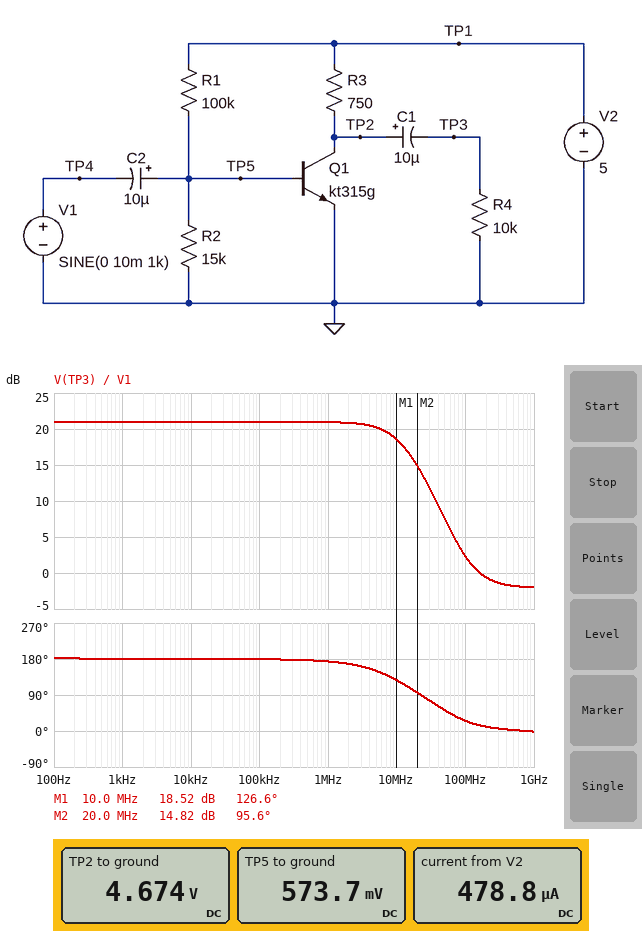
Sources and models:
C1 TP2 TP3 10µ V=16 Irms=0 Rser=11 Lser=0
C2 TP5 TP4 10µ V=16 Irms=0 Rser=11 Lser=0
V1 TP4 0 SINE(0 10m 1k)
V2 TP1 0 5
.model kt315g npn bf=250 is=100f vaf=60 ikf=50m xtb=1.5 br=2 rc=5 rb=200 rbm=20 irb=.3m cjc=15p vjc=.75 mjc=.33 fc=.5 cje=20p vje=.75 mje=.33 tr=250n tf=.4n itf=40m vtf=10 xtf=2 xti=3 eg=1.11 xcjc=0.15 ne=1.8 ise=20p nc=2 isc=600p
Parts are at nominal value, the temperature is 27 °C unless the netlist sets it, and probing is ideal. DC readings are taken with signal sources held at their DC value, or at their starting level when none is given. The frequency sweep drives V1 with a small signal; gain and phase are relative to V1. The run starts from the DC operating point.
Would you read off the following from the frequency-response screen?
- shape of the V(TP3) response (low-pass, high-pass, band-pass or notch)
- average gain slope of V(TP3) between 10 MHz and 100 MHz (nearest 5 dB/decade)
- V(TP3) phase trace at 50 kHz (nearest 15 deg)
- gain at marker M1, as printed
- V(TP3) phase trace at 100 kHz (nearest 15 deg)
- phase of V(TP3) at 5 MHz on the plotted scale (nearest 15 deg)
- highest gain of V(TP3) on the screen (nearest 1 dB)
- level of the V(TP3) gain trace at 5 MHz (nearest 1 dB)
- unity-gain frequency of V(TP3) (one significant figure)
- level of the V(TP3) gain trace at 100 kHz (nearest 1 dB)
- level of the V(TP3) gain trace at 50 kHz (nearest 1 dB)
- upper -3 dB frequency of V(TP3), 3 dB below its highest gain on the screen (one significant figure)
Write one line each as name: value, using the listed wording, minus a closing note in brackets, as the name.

shape of the V(TP3) response: low-pass
average gain slope of V(TP3) between 10 MHz and 100 MHz: -15 dB/decade
V(TP3) phase trace at 50 kHz: 180 deg
gain at marker M1, as printed: 18.52 dB
V(TP3) phase trace at 100 kHz: 180 deg
phase of V(TP3) at 5 MHz on the plotted scale: 150 deg
highest gain of V(TP3) on the screen: 21 dB
level of the V(TP3) gain trace at 5 MHz: 20 dB
unity-gain frequency of V(TP3): 200 MHz
level of the V(TP3) gain trace at 100 kHz: 21 dB
level of the V(TP3) gain trace at 50 kHz: 21 dB
upper -3 dB frequency of V(TP3), 3 dB below its highest gain on the screen: 10 MHz
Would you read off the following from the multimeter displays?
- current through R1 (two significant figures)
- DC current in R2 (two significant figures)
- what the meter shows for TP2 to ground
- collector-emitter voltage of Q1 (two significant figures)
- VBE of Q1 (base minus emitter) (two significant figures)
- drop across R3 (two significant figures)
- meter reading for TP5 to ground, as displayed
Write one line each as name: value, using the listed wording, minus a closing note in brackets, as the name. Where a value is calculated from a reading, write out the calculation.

current through R1: (5 V - 573.7 mV) / 100 kΩ = 44 µA
DC current in R2: (573.7 mV) / 15 kΩ = 38 µA
what the meter shows for TP2 to ground: 4.674 V
collector-emitter voltage of Q1: 4.674 V = 4.7 V
VBE of Q1 (base minus emitter): 573.7 mV = 570 mV
drop across R3: 5 V - 4.674 V = 330 mV
meter reading for TP5 to ground, as displayed: 573.7 mV
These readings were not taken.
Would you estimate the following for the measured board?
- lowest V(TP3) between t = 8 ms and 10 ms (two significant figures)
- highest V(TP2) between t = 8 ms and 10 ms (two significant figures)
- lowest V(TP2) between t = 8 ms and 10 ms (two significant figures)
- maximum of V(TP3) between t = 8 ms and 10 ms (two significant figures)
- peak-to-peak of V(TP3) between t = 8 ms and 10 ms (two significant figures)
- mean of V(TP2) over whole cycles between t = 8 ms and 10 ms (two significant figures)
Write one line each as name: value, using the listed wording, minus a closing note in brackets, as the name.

lowest V(TP3) between t = 8 ms and 10 ms: -130 mV
highest V(TP2) between t = 8 ms and 10 ms: 4.8 V
lowest V(TP2) between t = 8 ms and 10 ms: 4.5 V
maximum of V(TP3) between t = 8 ms and 10 ms: 96 mV
peak-to-peak of V(TP3) between t = 8 ms and 10 ms: 230 mV
mean of V(TP2) over whole cycles between t = 8 ms and 10 ms: 4.7 V
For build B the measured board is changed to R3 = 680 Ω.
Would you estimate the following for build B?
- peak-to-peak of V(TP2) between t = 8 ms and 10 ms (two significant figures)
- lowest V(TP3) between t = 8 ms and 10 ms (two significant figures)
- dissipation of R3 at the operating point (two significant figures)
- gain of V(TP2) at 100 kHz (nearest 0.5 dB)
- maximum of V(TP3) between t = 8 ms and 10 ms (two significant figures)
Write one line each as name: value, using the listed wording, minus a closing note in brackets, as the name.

peak-to-peak of V(TP2) between t = 8 ms and 10 ms: 210 mV
lowest V(TP3) between t = 8 ms and 10 ms: -120 mV
dissipation of R3 at the operating point: 130 µW
gain of V(TP2) at 100 kHz: 20.0 dB
maximum of V(TP3) between t = 8 ms and 10 ms: 88 mV
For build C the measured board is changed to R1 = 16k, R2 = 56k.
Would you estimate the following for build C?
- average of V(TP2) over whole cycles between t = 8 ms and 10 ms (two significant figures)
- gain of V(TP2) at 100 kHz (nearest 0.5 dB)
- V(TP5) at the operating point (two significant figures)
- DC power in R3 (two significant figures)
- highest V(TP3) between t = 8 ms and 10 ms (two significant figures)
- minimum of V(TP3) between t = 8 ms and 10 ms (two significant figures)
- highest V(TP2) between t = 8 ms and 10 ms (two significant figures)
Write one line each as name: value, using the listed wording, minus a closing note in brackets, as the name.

average of V(TP2) over whole cycles between t = 8 ms and 10 ms: 120 mV
gain of V(TP2) at 100 kHz: -1.0 dB
V(TP5) at the operating point: 680 mV
DC power in R3: 32 mW
highest V(TP3) between t = 8 ms and 10 ms: 15 mV
minimum of V(TP3) between t = 8 ms and 10 ms: -9.4 mV
highest V(TP2) between t = 8 ms and 10 ms: 130 mV
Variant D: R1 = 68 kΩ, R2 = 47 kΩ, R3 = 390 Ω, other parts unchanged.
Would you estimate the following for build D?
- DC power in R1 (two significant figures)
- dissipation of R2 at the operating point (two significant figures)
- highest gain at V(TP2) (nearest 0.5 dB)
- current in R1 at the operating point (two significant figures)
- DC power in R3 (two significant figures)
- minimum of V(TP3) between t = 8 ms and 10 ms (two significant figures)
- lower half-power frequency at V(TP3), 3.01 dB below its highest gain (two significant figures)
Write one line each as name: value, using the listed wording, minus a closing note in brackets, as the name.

DC power in R1: 280 µW
dissipation of R2 at the operating point: 9.1 µW
highest gain at V(TP2): 36.0 dB
current in R1 at the operating point: 64 µA
DC power in R3: 17 mW
minimum of V(TP3) between t = 8 ms and 10 ms: -690 mV
lower half-power frequency at V(TP3), 3.01 dB below its highest gain: 20 Hz
